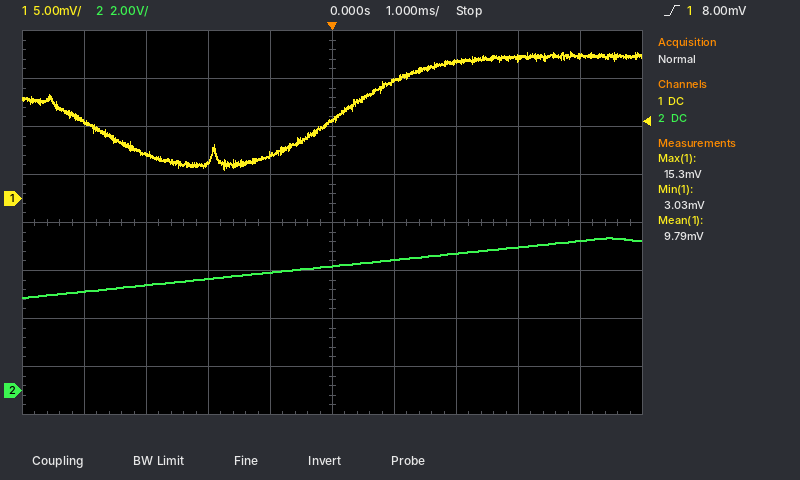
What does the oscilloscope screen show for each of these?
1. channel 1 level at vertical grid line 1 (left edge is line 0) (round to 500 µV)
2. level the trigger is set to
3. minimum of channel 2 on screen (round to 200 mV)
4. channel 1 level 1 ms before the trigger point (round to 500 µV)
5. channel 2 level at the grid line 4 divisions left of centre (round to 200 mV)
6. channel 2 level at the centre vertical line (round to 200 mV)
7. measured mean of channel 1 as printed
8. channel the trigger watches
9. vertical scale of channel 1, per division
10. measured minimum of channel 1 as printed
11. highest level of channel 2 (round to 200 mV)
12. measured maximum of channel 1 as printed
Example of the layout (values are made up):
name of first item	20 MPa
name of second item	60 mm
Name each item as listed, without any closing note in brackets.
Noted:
channel 1 level at vertical grid line 1 (left edge is line 0)	8.0 mV
level the trigger is set to	8.00 mV
minimum of channel 2 on screen	3.8 V
channel 1 level 1 ms before the trigger point	4.5 mV
channel 2 level at the grid line 4 divisions left of centre	4.2 V
channel 2 level at the centre vertical line	5.2 V
measured mean of channel 1 as printed	9.79 mV
channel the trigger watches	channel 1
vertical scale of channel 1, per division	5 mV
measured minimum of channel 1 as printed	3.03 mV
highest level of channel 2	6.4 V
measured maximum of channel 1 as printed	15.3 mV
